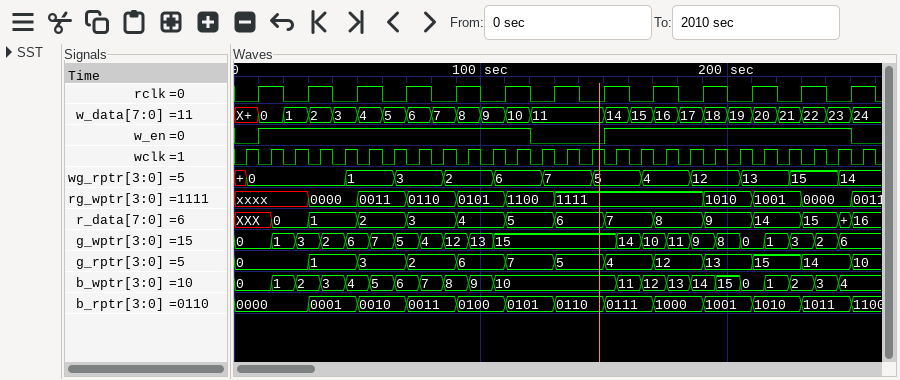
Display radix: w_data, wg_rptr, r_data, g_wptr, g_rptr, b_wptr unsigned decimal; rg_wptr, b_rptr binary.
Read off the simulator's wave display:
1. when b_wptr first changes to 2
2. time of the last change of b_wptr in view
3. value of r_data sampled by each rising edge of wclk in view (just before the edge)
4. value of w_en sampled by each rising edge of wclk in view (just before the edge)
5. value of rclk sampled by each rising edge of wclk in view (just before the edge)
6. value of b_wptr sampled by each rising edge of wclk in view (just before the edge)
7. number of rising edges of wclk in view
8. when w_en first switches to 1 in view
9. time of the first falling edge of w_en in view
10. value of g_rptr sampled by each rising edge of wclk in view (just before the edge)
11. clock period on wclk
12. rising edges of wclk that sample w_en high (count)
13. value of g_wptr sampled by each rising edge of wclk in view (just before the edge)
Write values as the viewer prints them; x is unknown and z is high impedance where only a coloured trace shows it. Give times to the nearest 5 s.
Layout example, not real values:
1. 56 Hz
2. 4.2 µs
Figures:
1. 25 s
2. 245 s
3. XXX, XXX, 0, 1, 1, 2, 2, 3, 3, 4, 4, 5, 5, 6, 6, 7, 7, 8, 8, 9, 9, 14, 14, 15, 15, 16
4. 0 1 1 1 1 1 1 1 1 1 1 1 0 0 0 1 1 1 1 1 1 1 1 1 1 0
5. 0 1 0 1 0 1 0 1 0 1 0 1 0 1 0 1 0 1 0 1 0 1 0 1 0 1
6. 0, 0, 1, 2, 3, 4, 5, 6, 7, 8, 9, 10, 10, 10, 10, 10, 11, 12, 13, 14, 15, 0, 1, 2, 3, 4
7. 26
8. 10 s
9. 120 s
10. 0, 0, 0, 1, 1, 3, 3, 2, 2, 6, 6, 7, 7, 5, 5, 4, 4, 12, 12, 13, 13, 15, 15, 14, 14, 10
11. 10 s
12. 21
13. 0, 0, 1, 3, 2, 6, 7, 5, 4, 12, 13, 15, 15, 15, 15, 15, 14, 10, 11, 9, 8, 0, 1, 3, 2, 6
